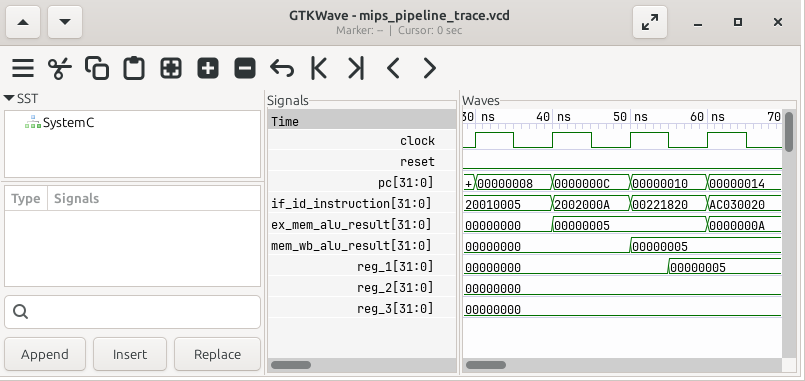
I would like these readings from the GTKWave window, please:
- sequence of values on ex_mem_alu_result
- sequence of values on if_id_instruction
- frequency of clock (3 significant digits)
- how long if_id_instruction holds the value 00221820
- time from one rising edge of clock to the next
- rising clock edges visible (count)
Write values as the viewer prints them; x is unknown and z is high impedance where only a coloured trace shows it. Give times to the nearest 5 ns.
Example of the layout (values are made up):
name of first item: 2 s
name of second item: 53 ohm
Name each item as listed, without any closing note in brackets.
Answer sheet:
sequence of values on ex_mem_alu_result: 00000000, 00000005, 0000000A
sequence of values on if_id_instruction: 20010005, 2002000A, 00221820, AC030020
frequency of clock: 100 MHz
how long if_id_instruction holds the value 00221820: 10 ns
time from one rising edge of clock to the next: 10 ns
rising clock edges visible: 4
